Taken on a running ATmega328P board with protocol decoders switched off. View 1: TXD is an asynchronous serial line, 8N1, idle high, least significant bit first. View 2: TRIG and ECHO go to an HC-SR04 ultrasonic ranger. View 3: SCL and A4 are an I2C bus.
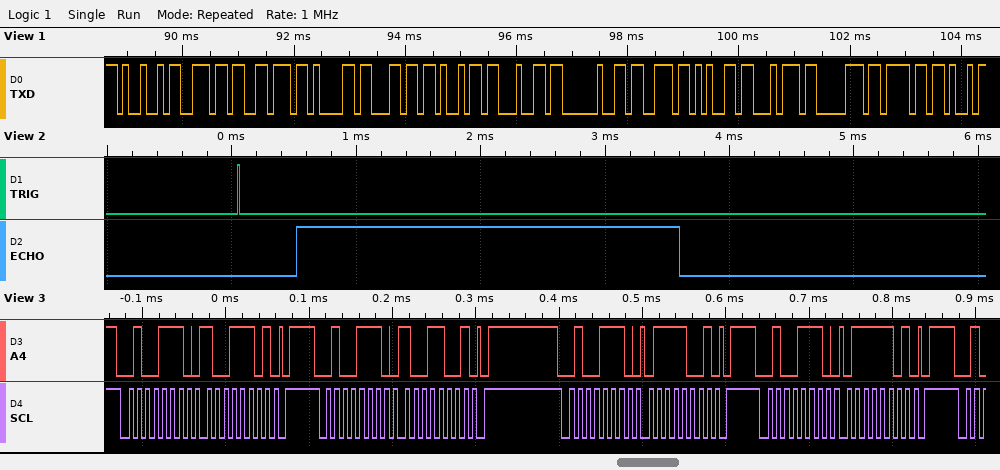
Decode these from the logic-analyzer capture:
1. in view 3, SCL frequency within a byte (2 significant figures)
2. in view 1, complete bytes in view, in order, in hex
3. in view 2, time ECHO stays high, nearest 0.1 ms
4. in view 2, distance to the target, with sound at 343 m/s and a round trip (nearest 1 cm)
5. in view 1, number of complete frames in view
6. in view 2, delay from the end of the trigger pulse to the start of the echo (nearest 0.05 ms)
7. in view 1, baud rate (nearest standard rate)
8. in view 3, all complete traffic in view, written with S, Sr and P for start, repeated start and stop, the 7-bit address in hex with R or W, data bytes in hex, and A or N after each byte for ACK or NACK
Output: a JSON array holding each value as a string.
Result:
["100 kHz", "0x49 0x6E 0x76 0x61 0x6C 0x69 0x64 0x20 0x73 0x65 0x74 0x70 0x6F", "3.1 ms", "53 cm", "13", "0.45 ms", "9600 baud", "S 27W A 9D A P S 27W A 99 A P S 27W A 79 A P S 27W A 7D A P"]
